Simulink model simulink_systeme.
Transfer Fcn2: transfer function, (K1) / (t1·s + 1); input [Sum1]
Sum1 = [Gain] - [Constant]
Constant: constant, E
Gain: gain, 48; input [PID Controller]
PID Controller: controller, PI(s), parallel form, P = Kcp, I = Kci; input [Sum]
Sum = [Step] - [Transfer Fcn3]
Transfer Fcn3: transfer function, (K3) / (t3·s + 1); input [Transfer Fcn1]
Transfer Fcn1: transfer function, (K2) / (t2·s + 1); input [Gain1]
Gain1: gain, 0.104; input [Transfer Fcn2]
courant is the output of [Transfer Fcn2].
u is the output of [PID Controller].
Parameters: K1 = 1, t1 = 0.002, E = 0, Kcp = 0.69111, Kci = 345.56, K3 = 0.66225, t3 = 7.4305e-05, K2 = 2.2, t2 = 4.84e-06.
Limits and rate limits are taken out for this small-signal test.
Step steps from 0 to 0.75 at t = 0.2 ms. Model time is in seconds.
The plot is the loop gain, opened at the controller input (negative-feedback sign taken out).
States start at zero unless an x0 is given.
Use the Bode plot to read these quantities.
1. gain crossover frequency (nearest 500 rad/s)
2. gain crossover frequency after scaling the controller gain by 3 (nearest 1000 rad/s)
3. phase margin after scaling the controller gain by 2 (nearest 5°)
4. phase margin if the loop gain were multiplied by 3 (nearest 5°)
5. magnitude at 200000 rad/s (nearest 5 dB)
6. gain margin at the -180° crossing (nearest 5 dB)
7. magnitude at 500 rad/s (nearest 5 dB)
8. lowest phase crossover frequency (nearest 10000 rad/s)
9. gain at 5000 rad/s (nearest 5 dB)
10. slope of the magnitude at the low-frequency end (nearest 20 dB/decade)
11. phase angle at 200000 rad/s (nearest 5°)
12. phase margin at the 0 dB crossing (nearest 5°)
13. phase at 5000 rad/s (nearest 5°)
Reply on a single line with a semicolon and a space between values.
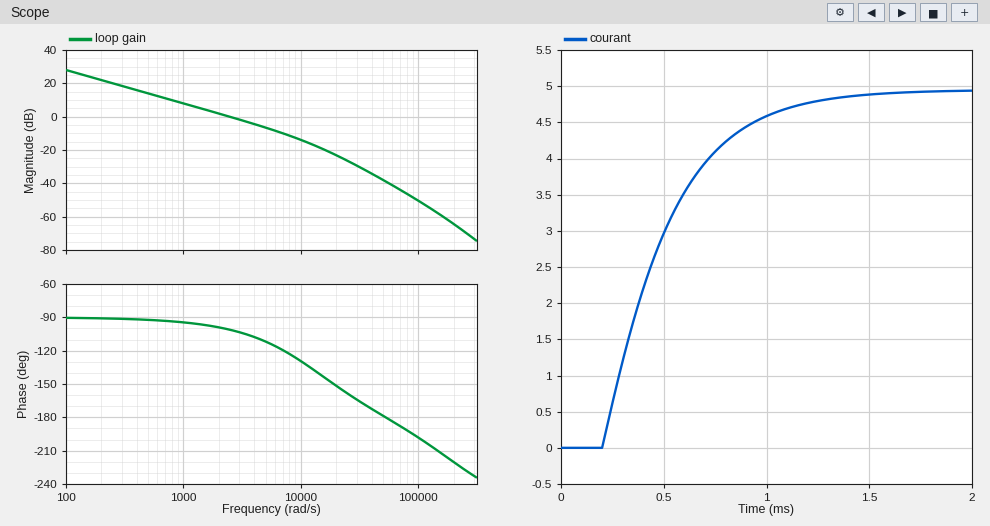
2500 rad/s; 7000 rad/s; 70°; 60°; -65 dB; 40 dB; 15 dB; 50000 rad/s; -5 dB; -20 dB/decade; -220°; 80°; -110°
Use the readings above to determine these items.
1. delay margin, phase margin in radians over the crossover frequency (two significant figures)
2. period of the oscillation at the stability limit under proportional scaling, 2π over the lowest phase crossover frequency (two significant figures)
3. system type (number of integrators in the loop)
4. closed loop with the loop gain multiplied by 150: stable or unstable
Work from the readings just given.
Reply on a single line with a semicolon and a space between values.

0.00056 s; 0.00013 s; 1; unstable
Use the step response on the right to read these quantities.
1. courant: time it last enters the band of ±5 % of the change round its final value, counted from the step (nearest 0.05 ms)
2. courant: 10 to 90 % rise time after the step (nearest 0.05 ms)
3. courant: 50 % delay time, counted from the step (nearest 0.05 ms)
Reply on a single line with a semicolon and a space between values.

0.90 ms; 0.65 ms; 0.25 ms
